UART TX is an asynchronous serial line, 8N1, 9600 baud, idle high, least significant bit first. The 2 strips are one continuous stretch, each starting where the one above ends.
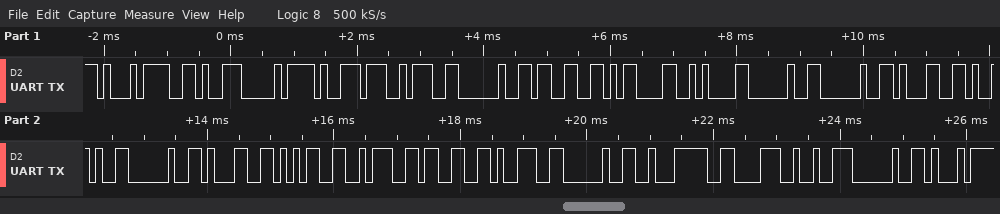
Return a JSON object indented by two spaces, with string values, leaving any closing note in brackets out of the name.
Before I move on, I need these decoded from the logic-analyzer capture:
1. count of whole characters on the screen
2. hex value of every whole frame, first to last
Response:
{
  "count of whole characters on the screen": "25",
  "hex value of every whole frame, first to last": "D1 96 D0 B9 3A 20 33 0D 0A 20 20 31 29 20 31 35 3A 33 39 20 E2 86 92 20 D1"
}
